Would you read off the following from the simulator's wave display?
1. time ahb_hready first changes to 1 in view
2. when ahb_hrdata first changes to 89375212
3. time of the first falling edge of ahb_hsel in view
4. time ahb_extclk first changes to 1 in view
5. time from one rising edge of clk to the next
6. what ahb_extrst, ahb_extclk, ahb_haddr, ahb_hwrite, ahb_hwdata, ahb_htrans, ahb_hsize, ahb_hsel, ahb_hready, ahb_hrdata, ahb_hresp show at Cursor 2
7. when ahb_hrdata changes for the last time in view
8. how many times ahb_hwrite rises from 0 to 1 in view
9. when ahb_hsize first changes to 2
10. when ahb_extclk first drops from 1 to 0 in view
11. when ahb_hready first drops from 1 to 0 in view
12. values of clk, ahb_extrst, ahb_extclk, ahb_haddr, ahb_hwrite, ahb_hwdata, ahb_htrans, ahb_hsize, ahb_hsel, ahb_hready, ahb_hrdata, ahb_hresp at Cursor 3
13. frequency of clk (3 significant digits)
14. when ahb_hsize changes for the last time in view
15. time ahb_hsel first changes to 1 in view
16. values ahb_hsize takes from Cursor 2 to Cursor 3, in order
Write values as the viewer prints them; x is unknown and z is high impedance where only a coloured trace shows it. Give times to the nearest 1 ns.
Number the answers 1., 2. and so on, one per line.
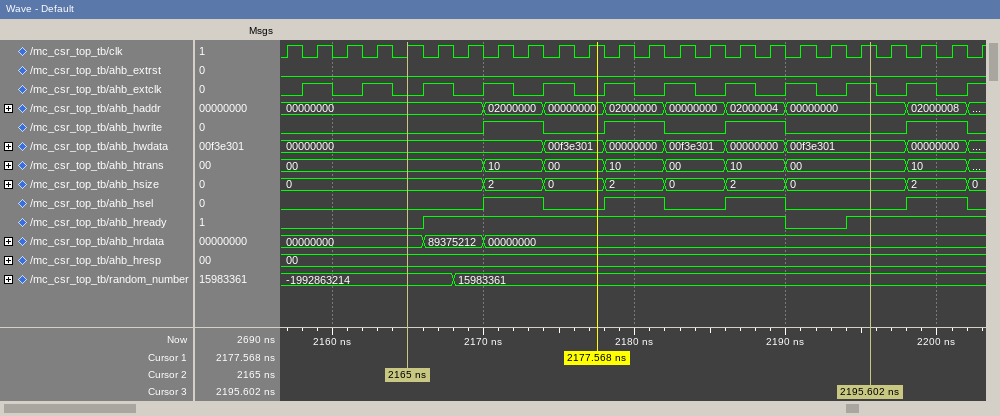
1. 2166 ns
2. 2166 ns
3. 2174 ns
4. 2158 ns
5. 2 ns
6. ahb_extrst=0, ahb_extclk=0, ahb_haddr=00000000, ahb_hwrite=0, ahb_hwdata=00000000, ahb_htrans=00, ahb_hsize=0, ahb_hsel=0, ahb_hready=0, ahb_hrdata=00000000, ahb_hresp=00
7. 2170 ns
8. 4
9. 2170 ns
10. 2160 ns
11. 2190 ns
12. clk=1, ahb_extrst=0, ahb_extclk=1, ahb_haddr=00000000, ahb_hwrite=0, ahb_hwdata=00f3e301, ahb_htrans=00, ahb_hsize=0, ahb_hsel=0, ahb_hready=1, ahb_hrdata=00000000, ahb_hresp=00
13. 500 MHz
14. 2202 ns
15. 2170 ns
16. 0, 2, 0, 2, 0, 2, 0
